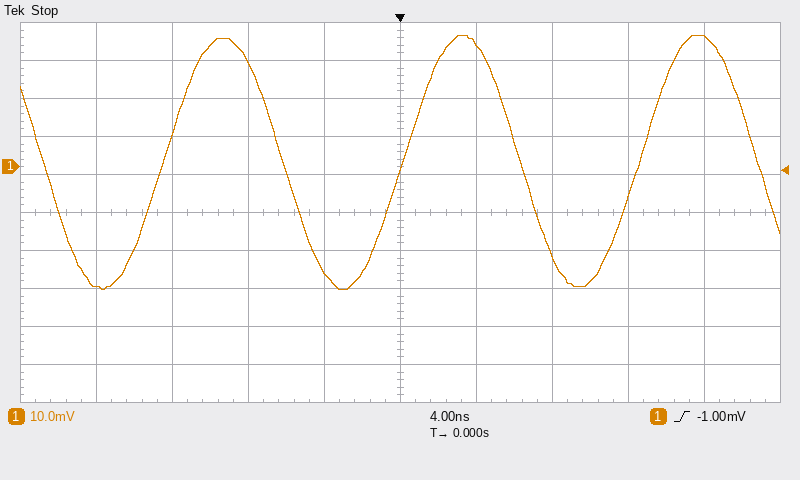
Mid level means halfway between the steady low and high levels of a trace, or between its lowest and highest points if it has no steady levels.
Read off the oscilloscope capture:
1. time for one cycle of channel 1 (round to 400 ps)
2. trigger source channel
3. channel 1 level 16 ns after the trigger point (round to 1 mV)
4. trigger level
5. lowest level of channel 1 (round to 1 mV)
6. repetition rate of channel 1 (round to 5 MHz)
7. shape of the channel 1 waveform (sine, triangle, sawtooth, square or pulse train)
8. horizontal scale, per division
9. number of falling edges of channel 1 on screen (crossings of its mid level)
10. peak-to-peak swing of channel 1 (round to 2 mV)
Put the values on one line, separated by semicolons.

12.4 ns; channel 1; 34 mV; -1.00 mV; -32 mV; 80 MHz; sine; 4 ns; 4; 66 mV
